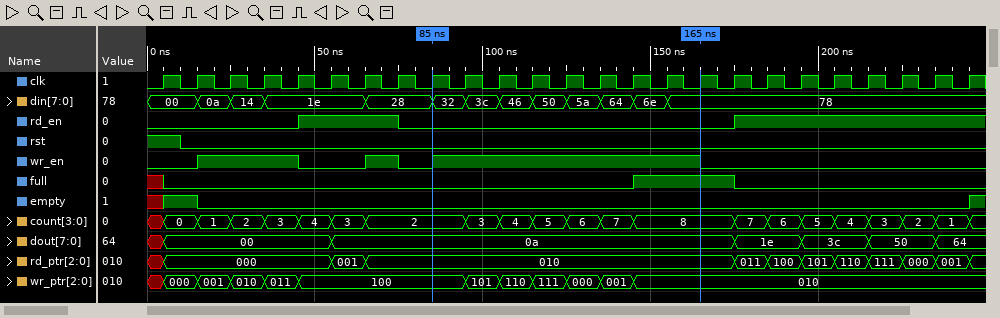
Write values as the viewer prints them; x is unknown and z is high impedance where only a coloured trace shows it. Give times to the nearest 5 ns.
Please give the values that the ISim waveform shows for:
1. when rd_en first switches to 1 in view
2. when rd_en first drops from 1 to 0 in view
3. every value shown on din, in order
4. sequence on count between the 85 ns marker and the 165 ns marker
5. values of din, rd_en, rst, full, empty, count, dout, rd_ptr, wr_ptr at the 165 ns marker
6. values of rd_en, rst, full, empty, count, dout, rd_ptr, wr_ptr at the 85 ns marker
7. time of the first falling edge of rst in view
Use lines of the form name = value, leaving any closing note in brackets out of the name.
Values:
when rd_en first switches to 1 in view = 45 ns
when rd_en first drops from 1 to 0 in view = 75 ns
every value shown on din, in order = 00, 0a, 14, 1e, 28, 32, 3c, 46, 50, 5a, 64, 6e, 78
sequence on count between the 85 ns marker and the 165 ns marker = 2, 3, 4, 5, 6, 7, 8
values of din, rd_en, rst, full, empty, count, dout, rd_ptr, wr_ptr at the 165 ns marker = din=78, rd_en=0, rst=0, full=1, empty=0, count=8, dout=0a, rd_ptr=010, wr_ptr=010
values of rd_en, rst, full, empty, count, dout, rd_ptr, wr_ptr at the 85 ns marker = rd_en=0, rst=0, full=0, empty=0, count=2, dout=0a, rd_ptr=010, wr_ptr=100
time of the first falling edge of rst in view = 10 ns
